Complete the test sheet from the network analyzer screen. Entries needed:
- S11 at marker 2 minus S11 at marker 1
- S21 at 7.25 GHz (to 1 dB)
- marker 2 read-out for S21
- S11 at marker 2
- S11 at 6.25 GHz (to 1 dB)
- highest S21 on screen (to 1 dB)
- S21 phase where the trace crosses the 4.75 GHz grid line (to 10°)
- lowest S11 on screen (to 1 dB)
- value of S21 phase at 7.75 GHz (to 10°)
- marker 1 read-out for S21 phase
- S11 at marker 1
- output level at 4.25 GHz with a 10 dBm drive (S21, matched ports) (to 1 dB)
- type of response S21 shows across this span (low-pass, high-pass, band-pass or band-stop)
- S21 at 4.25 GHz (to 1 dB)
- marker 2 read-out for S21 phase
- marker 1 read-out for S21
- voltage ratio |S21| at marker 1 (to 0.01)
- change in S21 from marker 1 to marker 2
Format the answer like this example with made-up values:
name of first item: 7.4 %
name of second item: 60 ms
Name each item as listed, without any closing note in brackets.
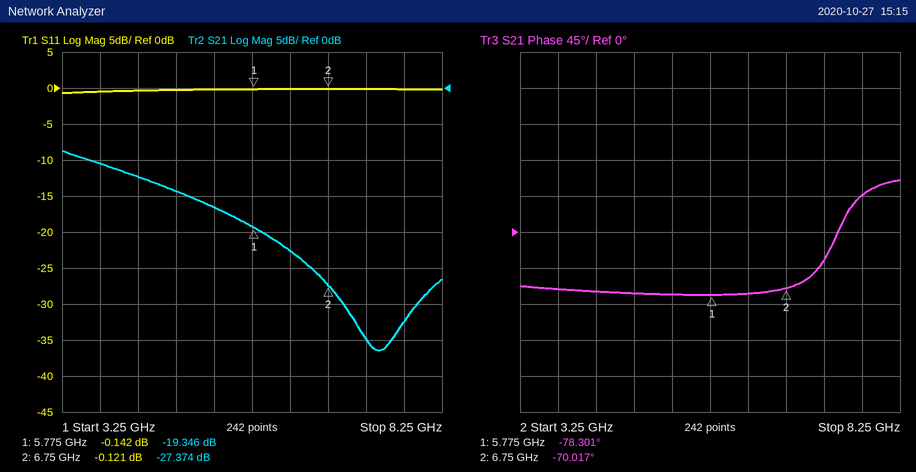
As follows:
S11 at marker 2 minus S11 at marker 1: 0.021 dB
S21 at 7.25 GHz: -35 dB
marker 2 read-out for S21: -27.374 dB
S11 at marker 2: -0.121 dB
S11 at 6.25 GHz: 0 dB
highest S21 on screen: -9 dB
S21 phase where the trace crosses the 4.75 GHz grid line: -80°
lowest S11 on screen: -1 dB
value of S21 phase at 7.75 GHz: 50°
marker 1 read-out for S21 phase: -78.301°
S11 at marker 1: -0.142 dB
output level at 4.25 GHz with a 10 dBm drive (S21, matched ports): -2 dBm
type of response S21 shows across this span: low-pass
S21 at 4.25 GHz: -12 dB
marker 2 read-out for S21 phase: -70.017°
marker 1 read-out for S21: -19.346 dB
voltage ratio |S21| at marker 1: 0.11
change in S21 from marker 1 to marker 2: -8.028 dB
